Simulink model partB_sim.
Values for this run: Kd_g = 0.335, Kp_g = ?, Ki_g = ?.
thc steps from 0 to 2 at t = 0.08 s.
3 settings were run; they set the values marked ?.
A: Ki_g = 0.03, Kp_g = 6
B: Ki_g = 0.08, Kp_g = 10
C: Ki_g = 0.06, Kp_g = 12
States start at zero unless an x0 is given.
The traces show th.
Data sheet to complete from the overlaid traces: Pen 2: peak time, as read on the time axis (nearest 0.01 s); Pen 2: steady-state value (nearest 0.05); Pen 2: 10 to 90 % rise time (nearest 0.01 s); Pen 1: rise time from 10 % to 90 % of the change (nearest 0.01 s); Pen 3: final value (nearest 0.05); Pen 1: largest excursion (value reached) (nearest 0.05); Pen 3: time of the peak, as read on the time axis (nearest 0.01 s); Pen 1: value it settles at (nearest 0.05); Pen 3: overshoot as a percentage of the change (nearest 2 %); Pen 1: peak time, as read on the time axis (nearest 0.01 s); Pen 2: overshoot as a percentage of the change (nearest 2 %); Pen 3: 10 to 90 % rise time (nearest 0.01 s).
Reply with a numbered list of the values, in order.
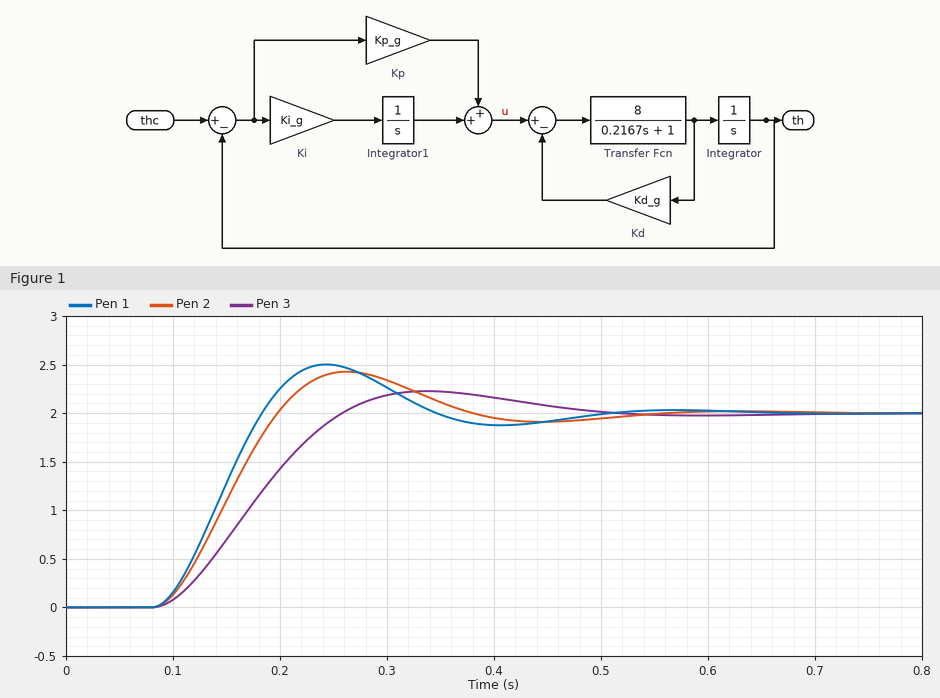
1. 0.26 s
2. 2.00
3. 0.08 s
4. 0.07 s
5. 2.00
6. 2.50
7. 0.34 s
8. 2.00
9. 12 %
10. 0.24 s
11. 22 %
12. 0.12 s
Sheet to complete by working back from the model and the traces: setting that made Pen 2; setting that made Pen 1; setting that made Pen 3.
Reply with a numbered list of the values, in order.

1. B
2. C
3. A
